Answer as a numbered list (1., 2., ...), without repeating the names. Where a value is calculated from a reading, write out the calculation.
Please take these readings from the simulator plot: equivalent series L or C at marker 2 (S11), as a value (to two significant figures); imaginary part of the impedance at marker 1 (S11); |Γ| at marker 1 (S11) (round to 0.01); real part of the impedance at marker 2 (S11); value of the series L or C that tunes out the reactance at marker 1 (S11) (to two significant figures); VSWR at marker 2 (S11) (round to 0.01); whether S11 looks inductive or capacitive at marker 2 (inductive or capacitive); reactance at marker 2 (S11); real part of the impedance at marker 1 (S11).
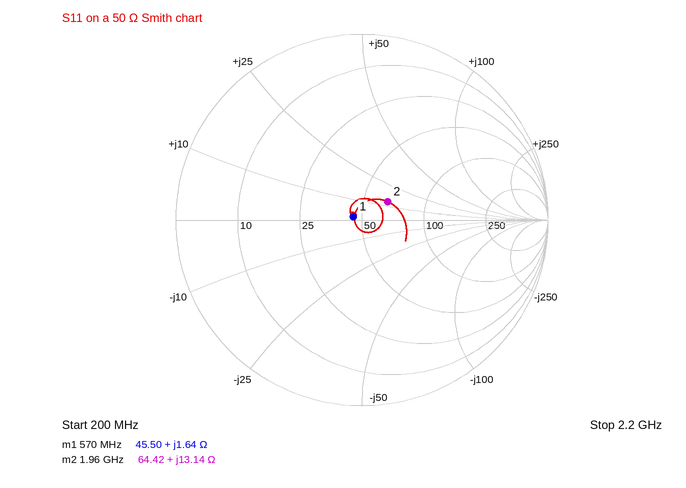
1. L = 13.14 Ω/(2π × 1.96 GHz) ≈ 1.1 nH
2. +1.64 Ω
3. 0.05
4. 64.42 Ω
5. C = 1/(2π × 570 MHz × 1.64 Ω) ≈ 170 pF
6. 1.41
7. inductive
8. +13.14 Ω
9. 45.50 Ω
